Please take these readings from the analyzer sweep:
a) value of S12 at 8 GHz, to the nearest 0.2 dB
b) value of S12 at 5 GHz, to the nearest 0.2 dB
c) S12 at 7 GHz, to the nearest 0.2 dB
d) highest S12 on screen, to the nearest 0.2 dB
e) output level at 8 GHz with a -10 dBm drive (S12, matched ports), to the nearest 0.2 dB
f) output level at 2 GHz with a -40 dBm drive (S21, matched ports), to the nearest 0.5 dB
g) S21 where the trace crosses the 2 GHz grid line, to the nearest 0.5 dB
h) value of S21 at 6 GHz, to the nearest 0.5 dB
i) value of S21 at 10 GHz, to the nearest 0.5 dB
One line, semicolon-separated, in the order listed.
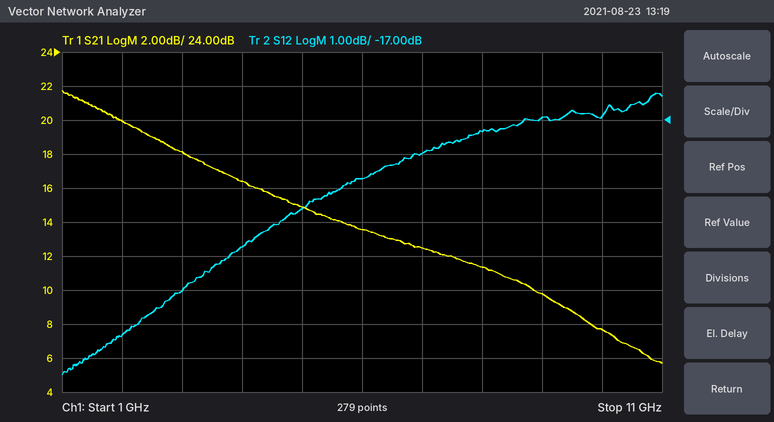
-17.4 dB; -19.6 dB; -18.0 dB; -16.2 dB; -27.4 dBm; -20.0 dBm; 20.0 dB; 13.5 dB; 7.5 dB
